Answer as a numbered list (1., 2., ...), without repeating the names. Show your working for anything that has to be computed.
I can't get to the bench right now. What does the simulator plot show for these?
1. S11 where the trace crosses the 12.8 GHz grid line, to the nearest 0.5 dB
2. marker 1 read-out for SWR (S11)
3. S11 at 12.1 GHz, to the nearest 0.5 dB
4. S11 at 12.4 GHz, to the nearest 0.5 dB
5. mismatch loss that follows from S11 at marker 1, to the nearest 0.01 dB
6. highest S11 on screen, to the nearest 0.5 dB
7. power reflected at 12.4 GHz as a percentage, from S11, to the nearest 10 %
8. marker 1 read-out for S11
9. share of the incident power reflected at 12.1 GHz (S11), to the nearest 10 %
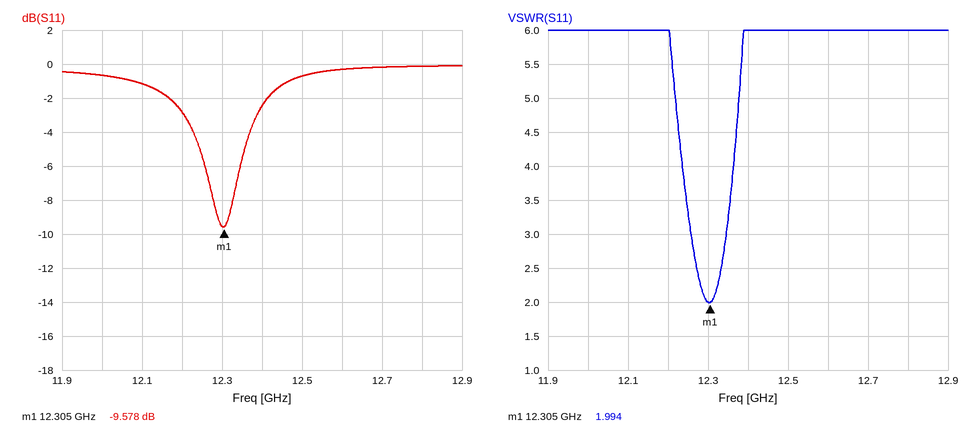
1. 0.0 dB
2. 1.994
3. -1.0 dB
4. -2.5 dB
5. −10 log10(1 − 10^(-9.578/10)) ≈ 0.51 dB
6. 0.0 dB
7. 10^(-2.5/10) ≈ 56.2 %, so 60 % to the nearest 10 %
8. -9.578 dB
9. 10^(-1/10) ≈ 79.4 %, so 80 % to the nearest 10 %
